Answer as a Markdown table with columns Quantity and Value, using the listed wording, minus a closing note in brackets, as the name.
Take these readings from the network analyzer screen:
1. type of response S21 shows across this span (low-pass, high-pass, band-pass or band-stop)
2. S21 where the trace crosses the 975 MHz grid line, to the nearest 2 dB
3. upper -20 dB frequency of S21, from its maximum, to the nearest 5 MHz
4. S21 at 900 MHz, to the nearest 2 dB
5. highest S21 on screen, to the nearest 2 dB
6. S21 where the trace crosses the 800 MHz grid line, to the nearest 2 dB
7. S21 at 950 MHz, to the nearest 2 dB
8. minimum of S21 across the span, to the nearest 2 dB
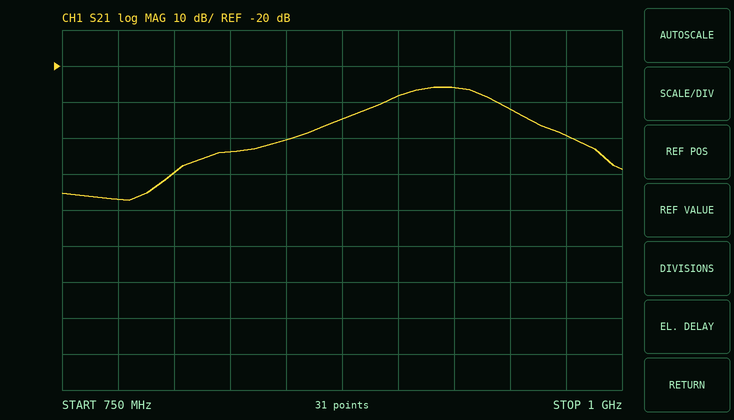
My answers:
| Quantity | Value |
|---|---|
| type of response S21 shows across this span | band-pass |
| S21 where the trace crosses the 975 MHz grid line, to the nearest 2 dB | -40 dB |
| upper -20 dB frequency of S21, from its maximum, to the nearest 5 MHz | 995 MHz |
| S21 at 900 MHz, to the nearest 2 dB | -28 dB |
| highest S21 on screen, to the nearest 2 dB | -26 dB |
| S21 where the trace crosses the 800 MHz grid line, to the nearest 2 dB | -50 dB |
| S21 at 950 MHz, to the nearest 2 dB | -32 dB |
| minimum of S21 across the span, to the nearest 2 dB | -58 dB |
